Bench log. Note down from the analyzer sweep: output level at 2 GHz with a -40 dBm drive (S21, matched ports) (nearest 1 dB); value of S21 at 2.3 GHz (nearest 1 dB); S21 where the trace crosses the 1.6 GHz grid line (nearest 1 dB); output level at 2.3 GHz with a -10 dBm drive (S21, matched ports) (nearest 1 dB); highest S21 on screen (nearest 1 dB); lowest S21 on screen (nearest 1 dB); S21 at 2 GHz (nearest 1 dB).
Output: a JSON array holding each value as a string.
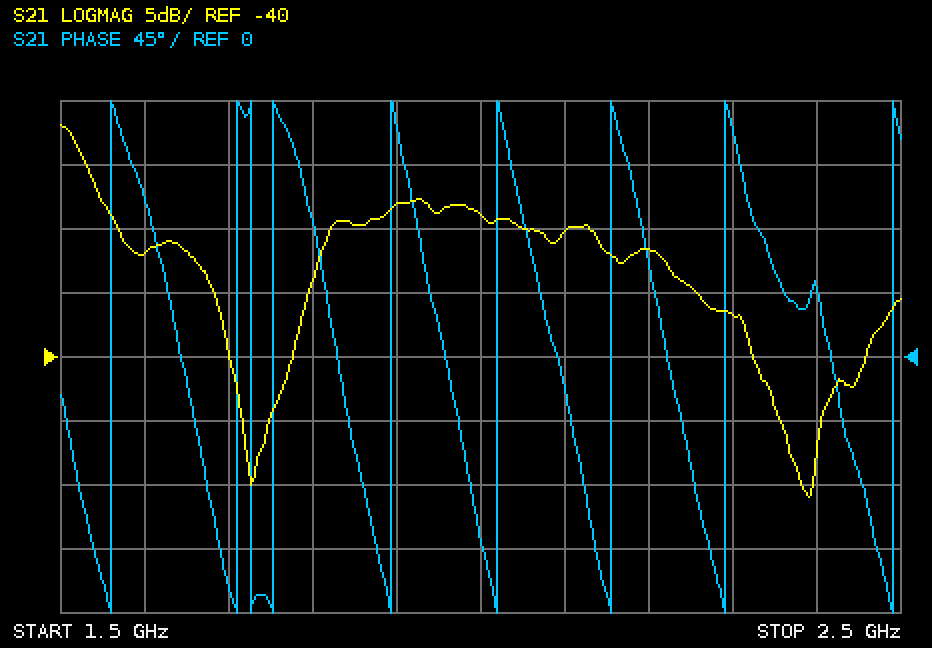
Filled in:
["-69 dBm", "-37 dB", "-32 dB", "-47 dBm", "-22 dB", "-51 dB", "-29 dB"]
